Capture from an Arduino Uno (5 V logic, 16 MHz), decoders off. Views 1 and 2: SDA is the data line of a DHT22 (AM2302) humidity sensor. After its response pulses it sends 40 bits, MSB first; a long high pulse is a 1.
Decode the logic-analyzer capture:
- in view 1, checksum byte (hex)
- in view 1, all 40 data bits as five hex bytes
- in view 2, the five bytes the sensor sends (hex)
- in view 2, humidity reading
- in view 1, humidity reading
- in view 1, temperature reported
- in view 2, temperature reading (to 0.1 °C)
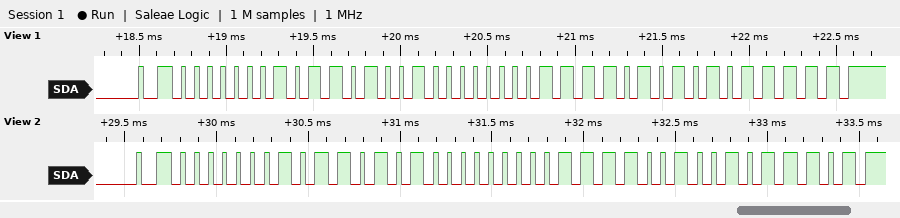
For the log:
0x5F
01 69 00 F5 5F
01 6A 00 F2 5D
36.2 %
36.1 %
24.5 °C
24.2 °C
